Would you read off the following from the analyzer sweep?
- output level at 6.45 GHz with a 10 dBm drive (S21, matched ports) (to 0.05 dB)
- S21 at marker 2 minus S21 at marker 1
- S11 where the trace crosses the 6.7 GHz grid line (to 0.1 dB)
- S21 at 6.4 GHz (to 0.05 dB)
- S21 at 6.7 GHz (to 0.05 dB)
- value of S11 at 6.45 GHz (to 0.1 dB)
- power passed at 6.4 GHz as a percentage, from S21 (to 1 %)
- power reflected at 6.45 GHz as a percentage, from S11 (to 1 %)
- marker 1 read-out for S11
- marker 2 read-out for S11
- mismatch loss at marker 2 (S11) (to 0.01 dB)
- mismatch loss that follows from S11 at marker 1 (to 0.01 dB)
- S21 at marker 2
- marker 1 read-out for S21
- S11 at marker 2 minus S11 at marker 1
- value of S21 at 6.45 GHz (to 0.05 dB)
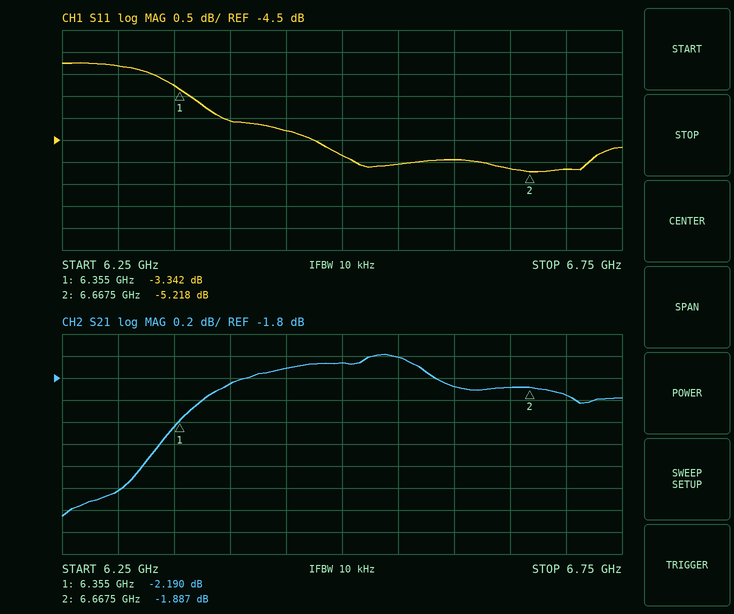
8.30 dBm
0.303 dB
-5.2 dB
-1.85 dB
-1.95 dB
-4.3 dB
65 %
37 %
-3.342 dB
-5.218 dB
1.55 dB
2.70 dB
-1.887 dB
-2.190 dB
-1.876 dB
-1.70 dB
